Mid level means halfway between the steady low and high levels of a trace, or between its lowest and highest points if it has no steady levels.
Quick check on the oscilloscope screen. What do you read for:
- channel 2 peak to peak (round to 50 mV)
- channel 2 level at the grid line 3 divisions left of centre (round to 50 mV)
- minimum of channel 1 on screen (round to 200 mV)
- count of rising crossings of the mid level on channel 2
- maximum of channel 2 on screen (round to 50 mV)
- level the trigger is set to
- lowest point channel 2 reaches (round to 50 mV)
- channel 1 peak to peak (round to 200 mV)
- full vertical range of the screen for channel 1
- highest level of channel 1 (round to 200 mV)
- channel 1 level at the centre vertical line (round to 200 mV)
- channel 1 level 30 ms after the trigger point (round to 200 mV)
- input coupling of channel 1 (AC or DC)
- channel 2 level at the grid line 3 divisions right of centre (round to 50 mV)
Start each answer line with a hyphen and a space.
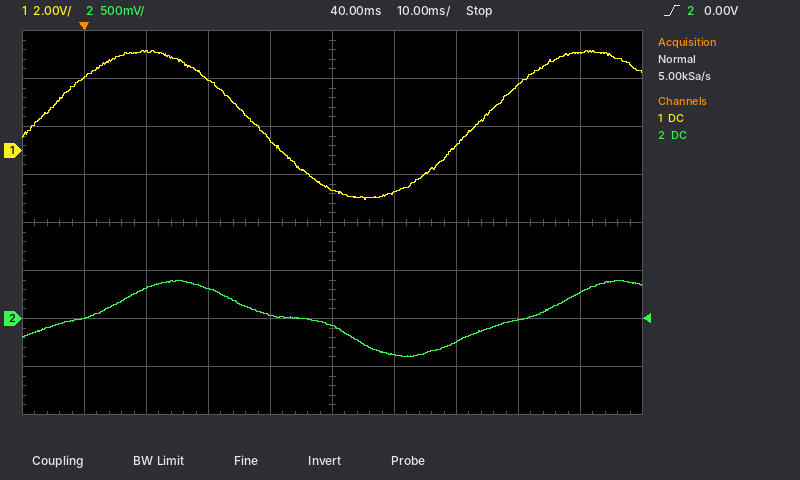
- 800 mV
- 300 mV
- -2.0 V
- 2
- 400 mV
- 0.00 V
- -400 mV
- 6.2 V
- 16 V
- 4.2 V
- -1.6 V
- 400 mV
- DC
- 0 mV
